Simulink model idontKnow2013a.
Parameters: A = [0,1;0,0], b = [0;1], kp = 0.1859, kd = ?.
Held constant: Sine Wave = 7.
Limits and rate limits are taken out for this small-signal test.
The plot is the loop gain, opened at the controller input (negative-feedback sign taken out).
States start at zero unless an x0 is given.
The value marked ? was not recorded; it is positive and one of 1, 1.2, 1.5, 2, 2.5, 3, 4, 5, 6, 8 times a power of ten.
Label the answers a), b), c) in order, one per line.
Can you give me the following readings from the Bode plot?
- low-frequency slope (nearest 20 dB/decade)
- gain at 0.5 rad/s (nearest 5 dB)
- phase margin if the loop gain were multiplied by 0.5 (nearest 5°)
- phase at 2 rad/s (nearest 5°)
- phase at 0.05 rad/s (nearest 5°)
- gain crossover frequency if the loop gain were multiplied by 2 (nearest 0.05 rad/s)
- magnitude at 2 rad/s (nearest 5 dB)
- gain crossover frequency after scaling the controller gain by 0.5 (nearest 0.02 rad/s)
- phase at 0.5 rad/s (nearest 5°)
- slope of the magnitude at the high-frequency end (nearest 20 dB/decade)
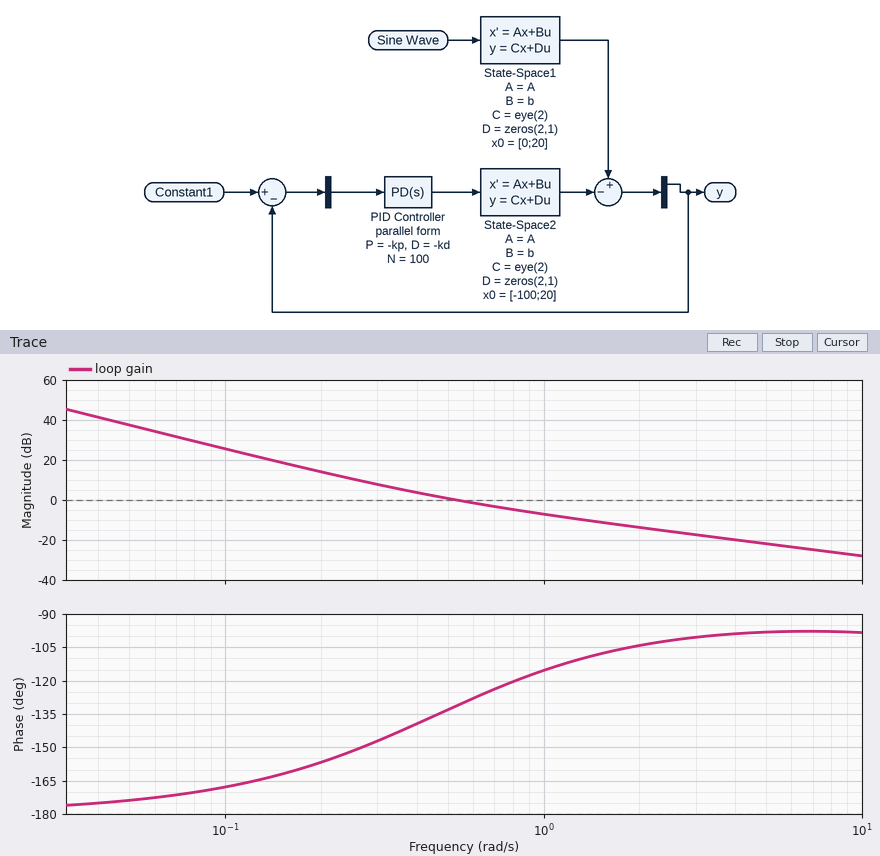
a) -40 dB/decade
b) 0 dB
c) 35°
d) -105°
e) -175°
f) 0.90 rad/s
g) -15 dB
h) 0.34 rad/s
i) -135°
j) -20 dB/decade
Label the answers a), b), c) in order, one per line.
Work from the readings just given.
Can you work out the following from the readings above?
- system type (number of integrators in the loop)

a) 2
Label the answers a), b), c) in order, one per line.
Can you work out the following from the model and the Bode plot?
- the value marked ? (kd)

a) 0.4
